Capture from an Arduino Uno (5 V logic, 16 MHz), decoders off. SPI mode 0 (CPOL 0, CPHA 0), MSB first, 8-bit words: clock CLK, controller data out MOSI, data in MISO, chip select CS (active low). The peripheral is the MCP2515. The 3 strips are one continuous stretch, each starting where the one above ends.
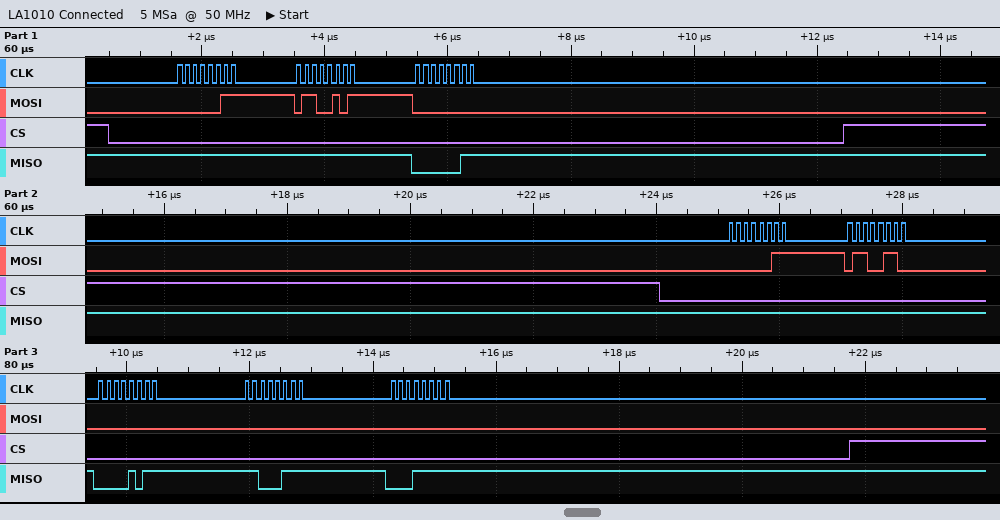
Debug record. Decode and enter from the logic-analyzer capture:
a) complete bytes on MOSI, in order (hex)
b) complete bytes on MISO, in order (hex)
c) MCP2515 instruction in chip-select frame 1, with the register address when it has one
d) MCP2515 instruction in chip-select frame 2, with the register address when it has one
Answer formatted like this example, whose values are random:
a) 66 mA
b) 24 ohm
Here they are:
a) 0x03 0x65 0x00 0x03 0x66 0x00 0x00 0x00
b) 0xFF 0xFF 0x03 0xFF 0xFF 0x0B 0xC7 0x1F
c) READ 0x65
d) READ 0x66
